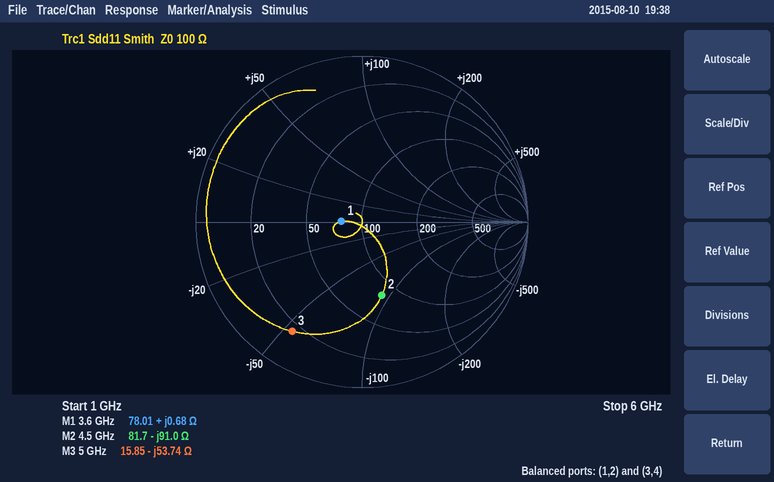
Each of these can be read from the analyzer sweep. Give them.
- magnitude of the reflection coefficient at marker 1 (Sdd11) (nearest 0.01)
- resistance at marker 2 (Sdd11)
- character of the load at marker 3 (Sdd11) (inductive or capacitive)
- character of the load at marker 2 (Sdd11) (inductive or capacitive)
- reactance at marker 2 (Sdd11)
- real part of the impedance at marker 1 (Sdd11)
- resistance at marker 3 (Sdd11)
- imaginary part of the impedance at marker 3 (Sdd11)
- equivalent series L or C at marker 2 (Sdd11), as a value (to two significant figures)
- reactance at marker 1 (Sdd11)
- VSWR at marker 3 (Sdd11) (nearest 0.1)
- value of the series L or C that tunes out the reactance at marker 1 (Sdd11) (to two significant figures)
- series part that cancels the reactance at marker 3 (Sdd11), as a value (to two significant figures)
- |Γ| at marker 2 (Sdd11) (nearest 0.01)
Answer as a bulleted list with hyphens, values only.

- 0.12
- 81.7 Ω
- capacitive
- capacitive
- -91.0 Ω
- 78.01 Ω
- 15.85 Ω
- -53.74 Ω
- 390 fF
- +0.68 Ω
- 8.2
- 65 pF
- 1.7 nH
- 0.46
